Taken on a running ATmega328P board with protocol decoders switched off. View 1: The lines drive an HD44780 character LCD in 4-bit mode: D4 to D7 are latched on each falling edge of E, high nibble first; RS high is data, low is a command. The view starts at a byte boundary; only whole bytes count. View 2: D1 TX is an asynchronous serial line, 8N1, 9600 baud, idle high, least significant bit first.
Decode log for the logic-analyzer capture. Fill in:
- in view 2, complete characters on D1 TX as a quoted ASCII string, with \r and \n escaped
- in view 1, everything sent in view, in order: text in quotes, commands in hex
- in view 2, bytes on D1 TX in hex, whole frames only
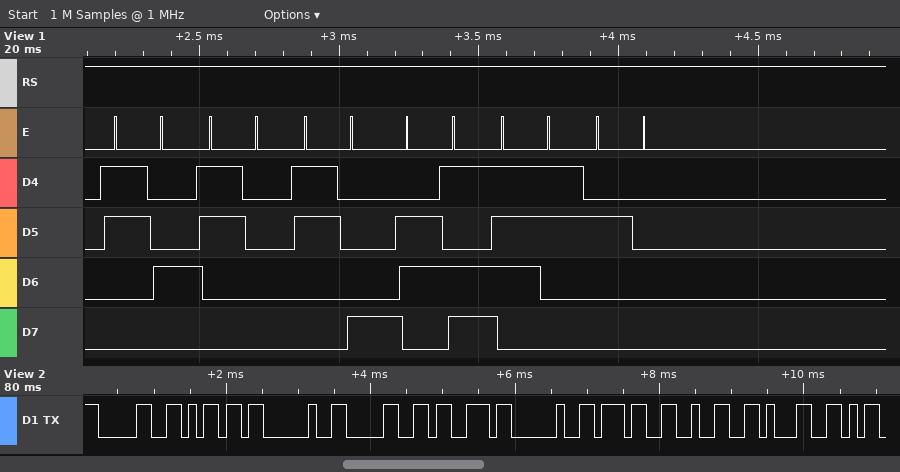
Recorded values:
"0m 0s 721"
"408ms "
30 6D 20 30 73 20 37 32 31
